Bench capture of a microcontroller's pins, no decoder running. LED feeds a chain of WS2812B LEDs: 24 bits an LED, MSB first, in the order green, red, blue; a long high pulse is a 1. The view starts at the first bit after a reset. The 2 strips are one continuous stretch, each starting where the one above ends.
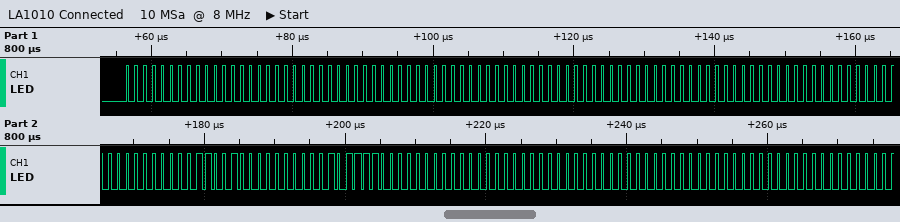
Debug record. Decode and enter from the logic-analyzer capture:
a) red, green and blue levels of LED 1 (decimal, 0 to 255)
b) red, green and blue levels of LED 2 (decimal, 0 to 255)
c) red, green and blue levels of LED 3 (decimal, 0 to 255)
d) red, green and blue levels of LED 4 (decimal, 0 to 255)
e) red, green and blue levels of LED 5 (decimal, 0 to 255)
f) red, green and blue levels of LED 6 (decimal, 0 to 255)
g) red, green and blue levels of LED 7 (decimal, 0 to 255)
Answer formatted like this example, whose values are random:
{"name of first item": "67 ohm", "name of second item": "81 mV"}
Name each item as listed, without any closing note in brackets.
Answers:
{"red, green and blue levels of LED 1": "0, 0, 0", "red, green and blue levels of LED 2": "0, 0, 0", "red, green and blue levels of LED 3": "0, 0, 0", "red, green and blue levels of LED 4": "0, 0, 0", "red, green and blue levels of LED 5": "0, 50, 94", "red, green and blue levels of LED 6": "0, 0, 0", "red, green and blue levels of LED 7": "0, 0, 0"}
